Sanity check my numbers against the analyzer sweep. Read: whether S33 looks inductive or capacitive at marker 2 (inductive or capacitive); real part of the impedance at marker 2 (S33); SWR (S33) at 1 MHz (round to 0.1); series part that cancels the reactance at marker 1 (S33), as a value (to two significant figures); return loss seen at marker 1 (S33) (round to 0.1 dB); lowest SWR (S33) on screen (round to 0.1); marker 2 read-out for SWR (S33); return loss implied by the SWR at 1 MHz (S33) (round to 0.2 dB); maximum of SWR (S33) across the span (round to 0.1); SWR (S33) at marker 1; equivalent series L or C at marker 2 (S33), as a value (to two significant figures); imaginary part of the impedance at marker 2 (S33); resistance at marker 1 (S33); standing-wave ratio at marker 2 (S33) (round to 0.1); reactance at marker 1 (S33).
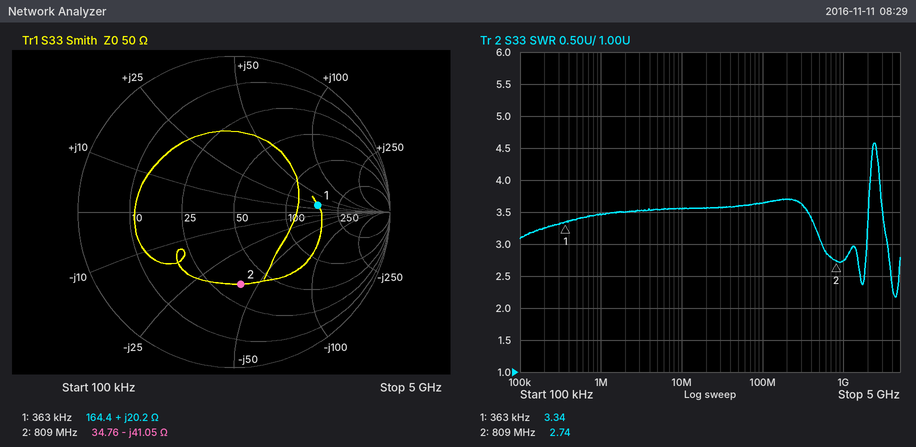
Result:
capacitive
34.76 Ω
3.5
22 nF
5.4 dB
2.2
2.74
5.2 dB
4.6
3.34
4.8 pF
-41.05 Ω
164.4 Ω
2.7
+20.2 Ω
